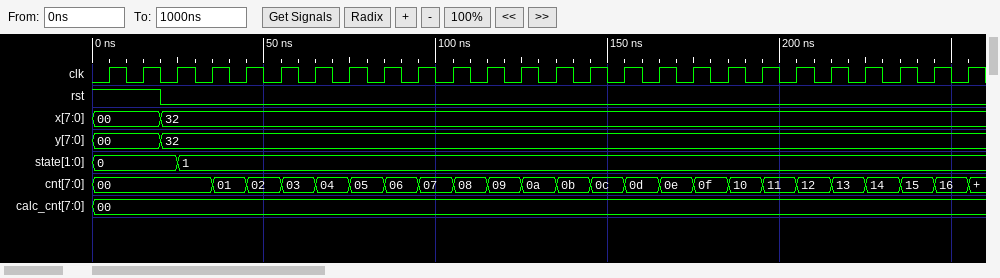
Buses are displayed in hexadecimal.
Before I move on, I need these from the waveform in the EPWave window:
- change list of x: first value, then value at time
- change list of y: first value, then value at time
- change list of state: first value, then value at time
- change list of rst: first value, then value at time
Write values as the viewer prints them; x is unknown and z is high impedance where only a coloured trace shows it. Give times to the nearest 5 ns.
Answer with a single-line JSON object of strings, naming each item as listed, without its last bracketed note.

{"change list of x: first value, then value at time": "00, 32 at 20 ns", "change list of y: first value, then value at time": "00, 32 at 20 ns", "change list of state: first value, then value at time": "0, 1 at 25 ns", "change list of rst: first value, then value at time": "1, 0 at 20 ns"}
